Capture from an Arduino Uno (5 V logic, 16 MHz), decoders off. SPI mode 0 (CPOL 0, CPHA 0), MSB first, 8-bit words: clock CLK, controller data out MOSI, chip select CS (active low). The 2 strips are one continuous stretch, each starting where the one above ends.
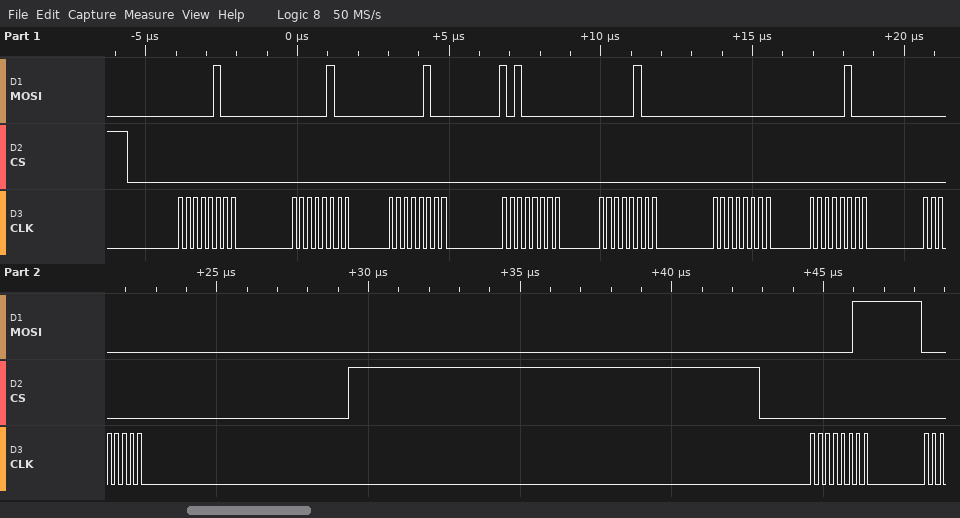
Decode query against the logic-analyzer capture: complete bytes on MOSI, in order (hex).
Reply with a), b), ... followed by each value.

a) 0x04 0x04 0x04 0xA0 0x04 0x00 0x04 0x00 0x03
